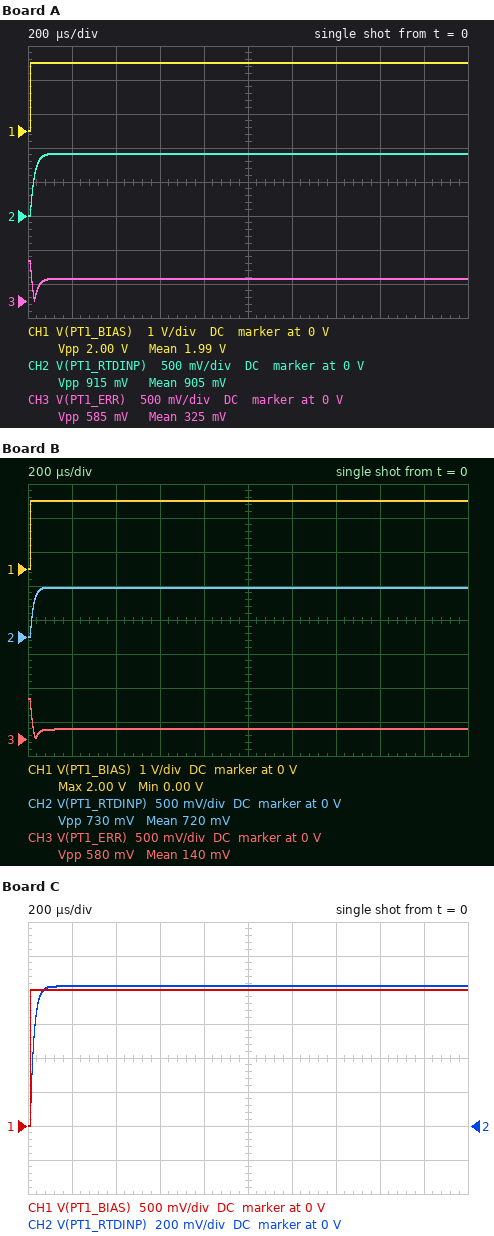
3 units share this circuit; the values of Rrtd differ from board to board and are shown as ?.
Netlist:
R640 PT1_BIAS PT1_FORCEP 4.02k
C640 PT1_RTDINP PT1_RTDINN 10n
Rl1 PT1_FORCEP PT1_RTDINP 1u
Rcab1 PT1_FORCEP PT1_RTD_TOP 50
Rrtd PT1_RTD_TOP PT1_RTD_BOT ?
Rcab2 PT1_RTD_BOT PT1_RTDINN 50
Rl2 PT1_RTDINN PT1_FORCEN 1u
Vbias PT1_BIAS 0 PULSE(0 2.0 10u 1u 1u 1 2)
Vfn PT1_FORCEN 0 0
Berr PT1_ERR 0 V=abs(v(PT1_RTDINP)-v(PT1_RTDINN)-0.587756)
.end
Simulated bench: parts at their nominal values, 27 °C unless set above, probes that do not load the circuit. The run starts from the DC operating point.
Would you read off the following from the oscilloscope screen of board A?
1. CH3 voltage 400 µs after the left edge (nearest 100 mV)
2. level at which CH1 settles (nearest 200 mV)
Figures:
300 mV
2.0 V
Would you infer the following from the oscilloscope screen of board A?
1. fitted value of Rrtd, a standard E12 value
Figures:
3.3 kΩ
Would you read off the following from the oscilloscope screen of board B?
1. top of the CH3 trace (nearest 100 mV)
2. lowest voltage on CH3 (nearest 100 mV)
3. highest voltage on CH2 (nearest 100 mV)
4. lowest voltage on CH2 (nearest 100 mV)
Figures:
600 mV
0 V
700 mV
0 V
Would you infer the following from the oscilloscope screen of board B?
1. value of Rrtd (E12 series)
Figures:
2.2 kΩ
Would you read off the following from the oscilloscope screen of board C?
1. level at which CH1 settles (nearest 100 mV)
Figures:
2.0 V
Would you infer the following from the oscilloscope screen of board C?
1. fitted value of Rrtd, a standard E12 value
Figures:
2.7 kΩ
